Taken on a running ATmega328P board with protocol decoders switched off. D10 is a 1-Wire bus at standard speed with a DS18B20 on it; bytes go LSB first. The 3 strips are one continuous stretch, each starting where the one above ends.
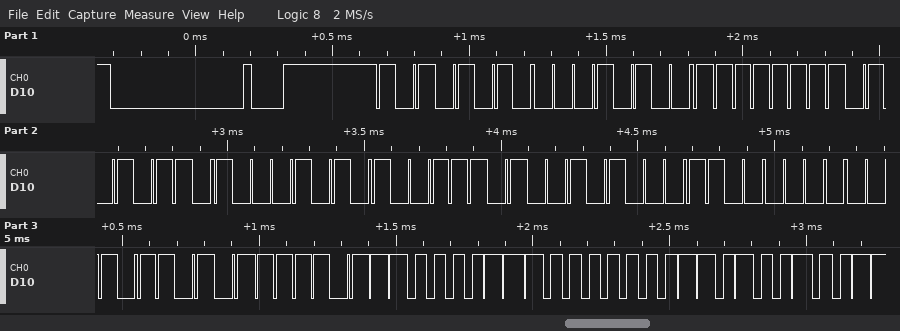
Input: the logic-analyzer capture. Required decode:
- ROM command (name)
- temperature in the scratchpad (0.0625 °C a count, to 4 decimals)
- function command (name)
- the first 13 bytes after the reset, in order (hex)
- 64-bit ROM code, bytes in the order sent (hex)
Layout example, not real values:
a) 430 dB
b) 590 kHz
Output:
a) Match ROM
b) 28.1875 °C
c) Read Scratchpad
d) 55 28 FF 6A 51 B9 14 03 B4 BE C3 01 4B
e) 28 FF 6A 51 B9 14 03 B4
